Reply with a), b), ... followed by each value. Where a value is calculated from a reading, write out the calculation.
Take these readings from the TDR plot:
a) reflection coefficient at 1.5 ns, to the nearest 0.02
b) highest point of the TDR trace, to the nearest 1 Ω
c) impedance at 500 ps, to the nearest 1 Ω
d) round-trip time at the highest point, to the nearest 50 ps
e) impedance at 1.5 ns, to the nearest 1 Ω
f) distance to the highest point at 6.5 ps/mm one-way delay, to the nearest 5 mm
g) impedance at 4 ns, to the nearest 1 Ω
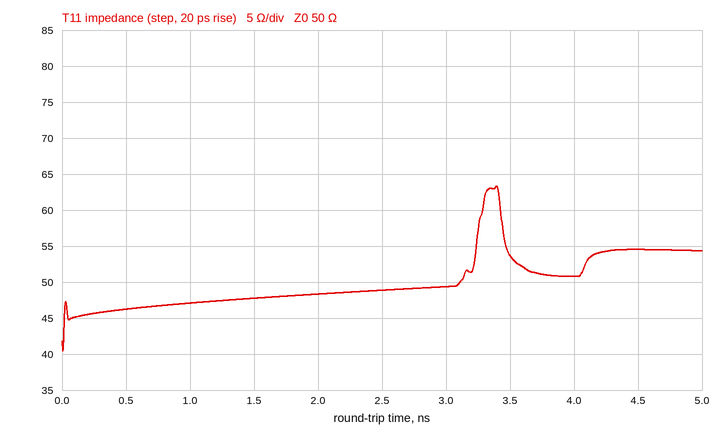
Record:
a) (48 − 50)/(48 + 50) ≈ -0.02
b) 63 Ω
c) 46 Ω
d) 3.40 ns
e) 48 Ω
f) 3.40 ns / 2 / 6.5 ps/mm ≈ 262 mm, so 260 mm to the nearest 5 mm
g) 51 Ω
